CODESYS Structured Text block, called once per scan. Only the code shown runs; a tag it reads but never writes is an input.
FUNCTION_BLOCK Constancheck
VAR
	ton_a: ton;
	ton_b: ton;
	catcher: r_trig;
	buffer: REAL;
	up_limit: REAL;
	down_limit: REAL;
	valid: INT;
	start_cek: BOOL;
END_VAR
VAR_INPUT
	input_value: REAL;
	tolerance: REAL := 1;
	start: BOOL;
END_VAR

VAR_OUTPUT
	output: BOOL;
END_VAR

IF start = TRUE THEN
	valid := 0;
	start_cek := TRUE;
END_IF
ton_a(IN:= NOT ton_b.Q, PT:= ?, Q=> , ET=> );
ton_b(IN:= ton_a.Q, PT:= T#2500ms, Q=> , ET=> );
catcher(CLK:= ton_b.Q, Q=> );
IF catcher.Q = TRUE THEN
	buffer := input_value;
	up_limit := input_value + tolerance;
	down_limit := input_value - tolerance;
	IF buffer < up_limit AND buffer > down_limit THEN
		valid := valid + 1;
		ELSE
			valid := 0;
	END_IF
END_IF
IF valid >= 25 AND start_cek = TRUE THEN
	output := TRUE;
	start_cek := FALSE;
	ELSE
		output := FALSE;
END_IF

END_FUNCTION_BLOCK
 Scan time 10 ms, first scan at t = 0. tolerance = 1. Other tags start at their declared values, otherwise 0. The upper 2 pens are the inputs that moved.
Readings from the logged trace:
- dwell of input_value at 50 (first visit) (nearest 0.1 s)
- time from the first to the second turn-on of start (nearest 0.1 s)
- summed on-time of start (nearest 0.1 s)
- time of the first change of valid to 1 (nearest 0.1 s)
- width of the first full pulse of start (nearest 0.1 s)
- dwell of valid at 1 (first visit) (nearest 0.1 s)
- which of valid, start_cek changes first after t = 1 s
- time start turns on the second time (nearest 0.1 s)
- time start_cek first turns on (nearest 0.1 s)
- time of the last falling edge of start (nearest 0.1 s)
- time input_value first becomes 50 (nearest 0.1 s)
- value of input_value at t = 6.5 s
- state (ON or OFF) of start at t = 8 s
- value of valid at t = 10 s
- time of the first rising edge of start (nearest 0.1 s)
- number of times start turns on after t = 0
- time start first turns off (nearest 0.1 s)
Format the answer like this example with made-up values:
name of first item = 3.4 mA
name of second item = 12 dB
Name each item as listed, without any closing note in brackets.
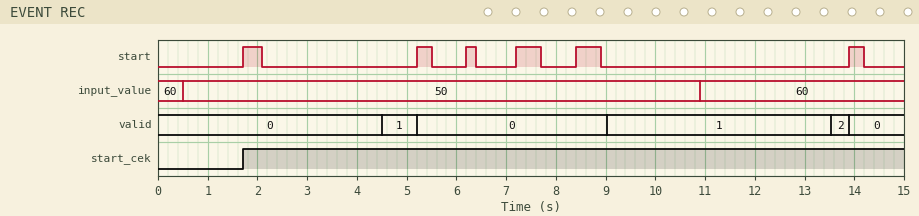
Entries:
dwell of input_value at 50 (first visit) = 10.4 s
time from the first to the second turn-on of start = 3.5 s
summed on-time of start = 2.2 s
time of the first change of valid to 1 = 4.5 s
width of the first full pulse of start = 0.4 s
dwell of valid at 1 (first visit) = 0.7 s
which of valid, start_cek changes first after t = 1 s = start_cek
time start turns on the second time = 5.2 s
time start_cek first turns on = 1.7 s
time of the last falling edge of start = 14.2 s
time input_value first becomes 50 = 0.5 s
value of input_value at t = 6.5 s = 50
state (ON or OFF) of start at t = 8 s = OFF
value of valid at t = 10 s = 1
time of the first rising edge of start = 1.7 s
number of times start turns on after t = 0 = 6
time start first turns off = 2.1 s
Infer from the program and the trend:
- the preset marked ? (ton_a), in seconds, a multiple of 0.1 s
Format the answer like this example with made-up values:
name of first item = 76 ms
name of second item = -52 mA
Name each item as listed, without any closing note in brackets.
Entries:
the preset marked ? (ton_a), in seconds, a multiple of 0.1 s = 2.0 s
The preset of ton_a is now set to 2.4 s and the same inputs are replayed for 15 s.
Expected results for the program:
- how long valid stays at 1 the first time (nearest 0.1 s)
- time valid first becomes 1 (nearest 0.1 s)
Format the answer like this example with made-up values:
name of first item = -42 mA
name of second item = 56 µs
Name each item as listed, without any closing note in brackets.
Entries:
how long valid stays at 1 the first time = 0.3 s
time valid first becomes 1 = 4.9 s
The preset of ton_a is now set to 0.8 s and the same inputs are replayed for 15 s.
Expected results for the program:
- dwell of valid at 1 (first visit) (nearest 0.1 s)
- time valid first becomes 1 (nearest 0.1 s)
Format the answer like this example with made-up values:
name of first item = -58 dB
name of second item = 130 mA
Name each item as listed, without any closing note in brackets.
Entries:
dwell of valid at 1 (first visit) = 1.9 s
time valid first becomes 1 = 3.3 s
